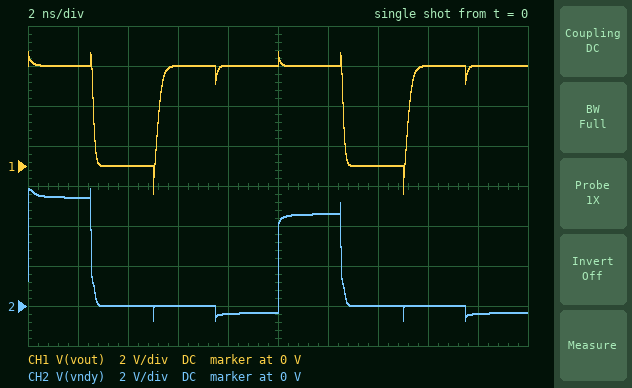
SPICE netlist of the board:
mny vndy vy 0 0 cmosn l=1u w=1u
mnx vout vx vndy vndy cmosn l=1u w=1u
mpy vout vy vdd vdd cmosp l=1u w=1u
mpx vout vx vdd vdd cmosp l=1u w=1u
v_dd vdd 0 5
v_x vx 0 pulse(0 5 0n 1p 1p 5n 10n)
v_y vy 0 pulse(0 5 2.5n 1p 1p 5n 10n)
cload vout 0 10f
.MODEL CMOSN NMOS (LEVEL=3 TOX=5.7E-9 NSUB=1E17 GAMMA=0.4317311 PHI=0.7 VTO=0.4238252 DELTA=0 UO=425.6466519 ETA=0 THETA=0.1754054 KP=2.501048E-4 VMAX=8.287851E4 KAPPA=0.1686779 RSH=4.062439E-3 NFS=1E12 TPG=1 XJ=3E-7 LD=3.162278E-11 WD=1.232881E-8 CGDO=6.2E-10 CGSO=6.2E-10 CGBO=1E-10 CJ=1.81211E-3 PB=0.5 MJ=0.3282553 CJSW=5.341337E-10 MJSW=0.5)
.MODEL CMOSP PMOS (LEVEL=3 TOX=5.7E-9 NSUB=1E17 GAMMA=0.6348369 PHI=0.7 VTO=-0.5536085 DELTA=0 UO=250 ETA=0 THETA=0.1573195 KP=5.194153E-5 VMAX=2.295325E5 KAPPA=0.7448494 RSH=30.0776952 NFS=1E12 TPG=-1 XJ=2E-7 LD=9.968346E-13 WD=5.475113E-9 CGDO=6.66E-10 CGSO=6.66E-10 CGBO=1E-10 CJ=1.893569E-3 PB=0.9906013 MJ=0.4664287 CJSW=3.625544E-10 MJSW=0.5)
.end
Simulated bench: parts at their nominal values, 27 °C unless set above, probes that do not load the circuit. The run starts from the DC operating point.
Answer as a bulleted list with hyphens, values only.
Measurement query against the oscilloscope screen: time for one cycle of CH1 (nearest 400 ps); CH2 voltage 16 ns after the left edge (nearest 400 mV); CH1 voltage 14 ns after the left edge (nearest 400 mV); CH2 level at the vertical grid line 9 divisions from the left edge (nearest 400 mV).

- 10.0 ns
- 0 V
- 0 V
- -400 mV
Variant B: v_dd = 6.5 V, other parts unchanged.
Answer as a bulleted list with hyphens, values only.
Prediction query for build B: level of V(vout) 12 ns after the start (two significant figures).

- 6.5 V
